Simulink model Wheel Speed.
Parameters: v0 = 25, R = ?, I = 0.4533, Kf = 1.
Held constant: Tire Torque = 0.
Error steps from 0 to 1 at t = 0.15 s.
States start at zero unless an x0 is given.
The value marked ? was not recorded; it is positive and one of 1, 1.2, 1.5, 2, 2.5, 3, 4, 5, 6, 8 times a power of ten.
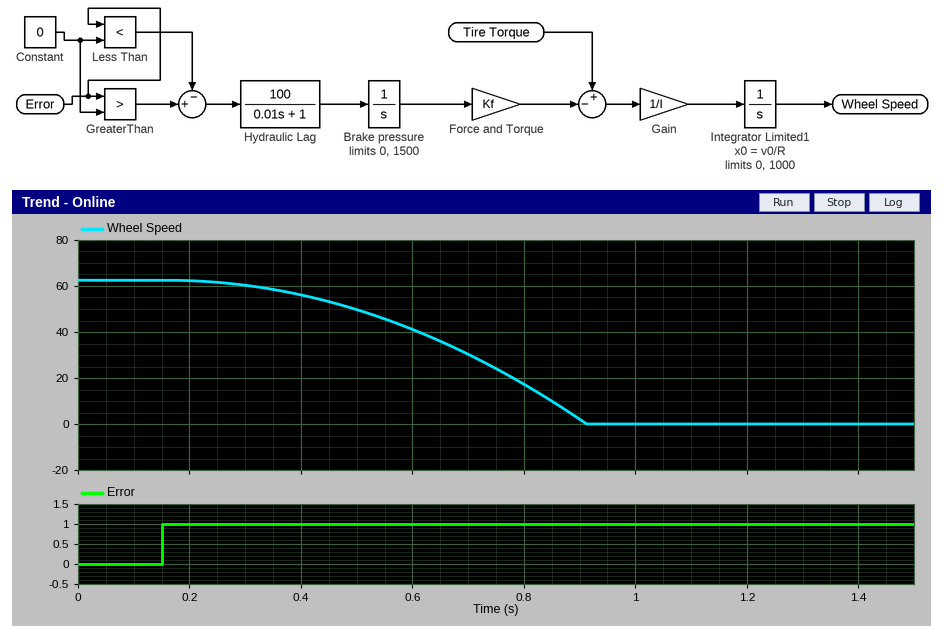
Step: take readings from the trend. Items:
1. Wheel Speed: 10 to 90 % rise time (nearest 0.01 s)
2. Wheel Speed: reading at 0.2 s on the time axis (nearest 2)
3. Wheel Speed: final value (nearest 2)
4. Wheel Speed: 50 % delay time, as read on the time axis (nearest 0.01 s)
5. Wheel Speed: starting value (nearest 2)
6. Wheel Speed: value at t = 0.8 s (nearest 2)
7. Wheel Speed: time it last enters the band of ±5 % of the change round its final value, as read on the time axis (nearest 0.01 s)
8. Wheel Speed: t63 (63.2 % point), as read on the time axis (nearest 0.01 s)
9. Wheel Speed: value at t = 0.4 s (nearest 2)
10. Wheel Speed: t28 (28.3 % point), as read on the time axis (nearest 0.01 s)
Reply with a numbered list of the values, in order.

1. 0.48 s
2. 62
3. 0
4. 0.69 s
5. 62
6. 18
7. 0.89 s
8. 0.76 s
9. 56
10. 0.56 s
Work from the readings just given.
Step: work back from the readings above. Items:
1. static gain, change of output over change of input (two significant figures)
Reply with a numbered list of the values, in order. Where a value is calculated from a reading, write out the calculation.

1. (0 - 62) / (1 - 0) = -62
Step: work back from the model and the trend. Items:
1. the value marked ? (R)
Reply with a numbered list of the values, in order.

1. 0.4
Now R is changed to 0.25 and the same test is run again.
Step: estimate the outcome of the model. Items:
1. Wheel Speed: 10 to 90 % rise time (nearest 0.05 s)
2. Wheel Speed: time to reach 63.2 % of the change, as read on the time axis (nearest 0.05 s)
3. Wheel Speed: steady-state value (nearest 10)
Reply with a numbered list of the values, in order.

1. 0.60 s
2. 0.90 s
3. 0
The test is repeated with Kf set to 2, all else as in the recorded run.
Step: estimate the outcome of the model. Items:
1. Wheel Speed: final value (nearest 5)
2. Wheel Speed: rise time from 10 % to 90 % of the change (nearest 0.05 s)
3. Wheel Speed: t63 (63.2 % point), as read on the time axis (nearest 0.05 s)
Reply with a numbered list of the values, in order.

1. 0
2. 0.35 s
3. 0.60 s
